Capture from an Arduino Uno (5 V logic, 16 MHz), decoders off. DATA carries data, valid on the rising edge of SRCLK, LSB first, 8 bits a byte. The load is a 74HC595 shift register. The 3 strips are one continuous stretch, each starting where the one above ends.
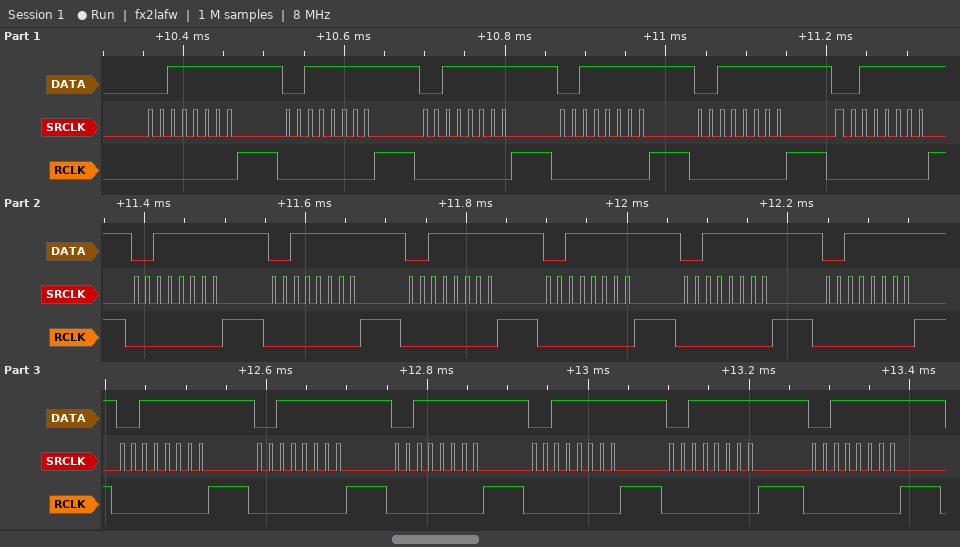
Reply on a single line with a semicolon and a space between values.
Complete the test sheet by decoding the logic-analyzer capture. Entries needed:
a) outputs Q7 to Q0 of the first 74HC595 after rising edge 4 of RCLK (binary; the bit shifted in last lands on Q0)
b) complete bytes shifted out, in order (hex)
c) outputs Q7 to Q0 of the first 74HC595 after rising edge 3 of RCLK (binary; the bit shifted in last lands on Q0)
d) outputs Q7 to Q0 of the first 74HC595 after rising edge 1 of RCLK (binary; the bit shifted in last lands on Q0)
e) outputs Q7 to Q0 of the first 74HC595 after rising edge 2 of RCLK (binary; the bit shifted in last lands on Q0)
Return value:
00111111; FC FC FC FC FC FC FC FC FC FC FC FC FC FC FC FC FC FC; 00111111; 00111111; 00111111
